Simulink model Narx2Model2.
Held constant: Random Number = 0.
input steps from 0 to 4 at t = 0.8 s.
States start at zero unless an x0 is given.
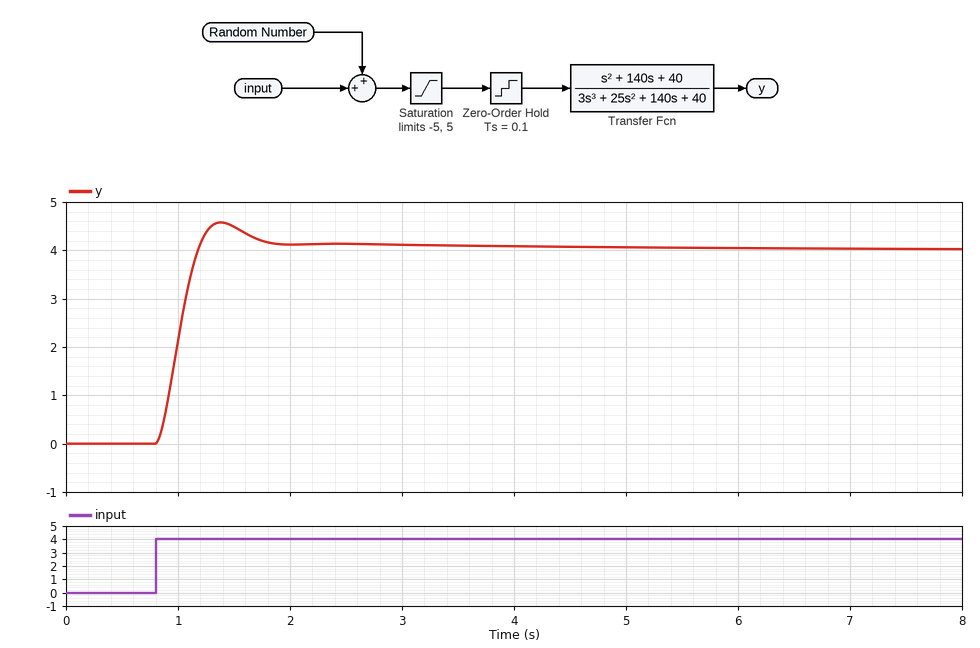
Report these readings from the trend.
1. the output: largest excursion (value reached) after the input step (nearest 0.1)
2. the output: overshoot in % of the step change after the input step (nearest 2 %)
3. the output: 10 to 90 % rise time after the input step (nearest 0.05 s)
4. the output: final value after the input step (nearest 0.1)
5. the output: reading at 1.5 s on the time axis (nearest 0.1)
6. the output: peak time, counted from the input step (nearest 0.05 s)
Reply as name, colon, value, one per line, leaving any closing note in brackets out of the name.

the output: largest excursion (value reached) after the input step: 4.6
the output: overshoot in % of the step change after the input step: 14 %
the output: 10 to 90 % rise time after the input step: 0.25 s
the output: final value after the input step: 4.0
the output: reading at 1.5 s on the time axis: 4.5
the output: peak time, counted from the input step: 0.60 s
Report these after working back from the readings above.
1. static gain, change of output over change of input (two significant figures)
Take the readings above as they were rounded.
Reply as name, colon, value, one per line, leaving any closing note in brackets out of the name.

static gain, change of output over change of input: 1.0
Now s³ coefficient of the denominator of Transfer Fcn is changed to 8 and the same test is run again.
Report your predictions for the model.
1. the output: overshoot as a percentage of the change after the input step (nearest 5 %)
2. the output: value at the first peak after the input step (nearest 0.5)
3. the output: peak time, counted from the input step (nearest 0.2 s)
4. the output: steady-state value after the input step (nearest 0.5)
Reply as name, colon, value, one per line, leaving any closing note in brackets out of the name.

the output: overshoot as a percentage of the change after the input step: 35 %
the output: value at the first peak after the input step: 5.5
the output: peak time, counted from the input step: 0.8 s
the output: steady-state value after the input step: 4.0
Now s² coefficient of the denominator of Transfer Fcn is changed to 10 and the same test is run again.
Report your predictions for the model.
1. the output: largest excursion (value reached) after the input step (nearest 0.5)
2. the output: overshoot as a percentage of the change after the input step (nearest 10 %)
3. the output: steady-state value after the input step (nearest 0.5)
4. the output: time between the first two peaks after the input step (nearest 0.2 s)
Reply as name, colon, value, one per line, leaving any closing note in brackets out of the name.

the output: largest excursion (value reached) after the input step: 6.0
the output: overshoot as a percentage of the change after the input step: 50 %
the output: steady-state value after the input step: 4.0
the output: time between the first two peaks after the input step: 1.0 s
